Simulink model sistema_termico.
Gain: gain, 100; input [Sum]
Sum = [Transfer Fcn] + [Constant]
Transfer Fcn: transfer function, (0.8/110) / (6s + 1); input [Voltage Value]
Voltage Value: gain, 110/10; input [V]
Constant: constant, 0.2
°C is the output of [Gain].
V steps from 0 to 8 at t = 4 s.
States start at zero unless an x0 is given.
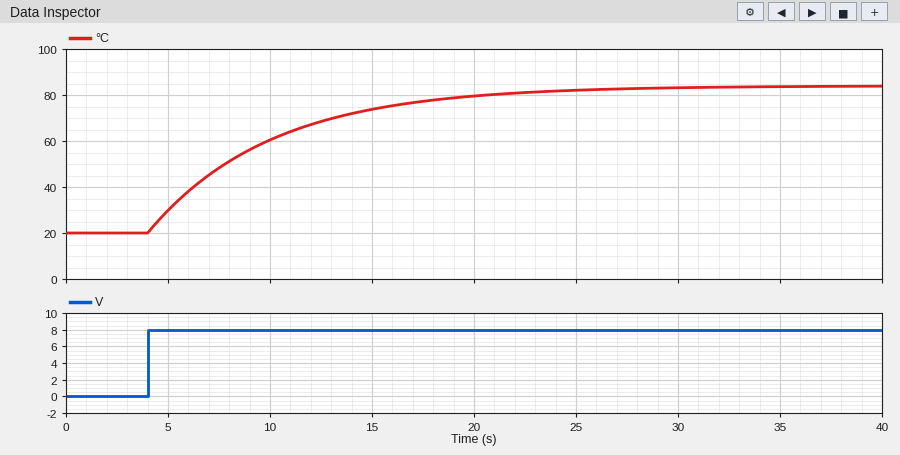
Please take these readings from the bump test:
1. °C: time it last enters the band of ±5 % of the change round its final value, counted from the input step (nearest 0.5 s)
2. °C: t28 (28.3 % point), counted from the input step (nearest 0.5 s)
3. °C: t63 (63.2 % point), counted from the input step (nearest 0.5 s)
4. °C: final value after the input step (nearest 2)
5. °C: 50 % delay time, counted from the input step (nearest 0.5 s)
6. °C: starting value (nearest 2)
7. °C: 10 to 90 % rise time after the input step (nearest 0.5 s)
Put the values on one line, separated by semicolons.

18.0 s; 2.0 s; 6.0 s; 84; 4.0 s; 20; 13.0 s
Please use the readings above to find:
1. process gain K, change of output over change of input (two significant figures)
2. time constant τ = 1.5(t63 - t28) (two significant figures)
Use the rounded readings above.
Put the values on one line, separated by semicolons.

8.0; 6.0 s
